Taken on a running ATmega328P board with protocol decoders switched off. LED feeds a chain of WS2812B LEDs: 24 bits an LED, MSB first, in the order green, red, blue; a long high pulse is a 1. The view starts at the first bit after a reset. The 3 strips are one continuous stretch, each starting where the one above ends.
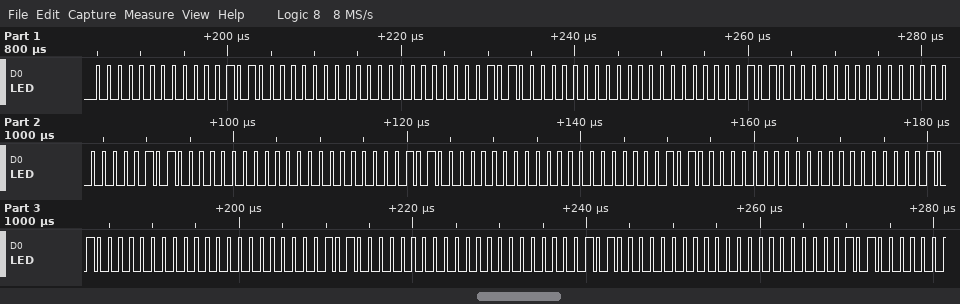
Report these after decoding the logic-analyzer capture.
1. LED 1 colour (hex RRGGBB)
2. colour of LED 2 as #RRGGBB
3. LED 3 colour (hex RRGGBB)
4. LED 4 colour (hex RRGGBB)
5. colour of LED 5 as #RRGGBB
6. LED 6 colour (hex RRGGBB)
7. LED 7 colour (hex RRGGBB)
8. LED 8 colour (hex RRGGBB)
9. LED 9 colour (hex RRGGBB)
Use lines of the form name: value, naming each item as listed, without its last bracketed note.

LED 1 colour: #0A0000
colour of LED 2 as #RRGGBB: #0A0000
LED 3 colour: #0A0000
LED 4 colour: #0A0000
colour of LED 5 as #RRGGBB: #0A0000
LED 6 colour: #0A0000
LED 7 colour: #0A0000
LED 8 colour: #0A0000
LED 9 colour: #0A0000
